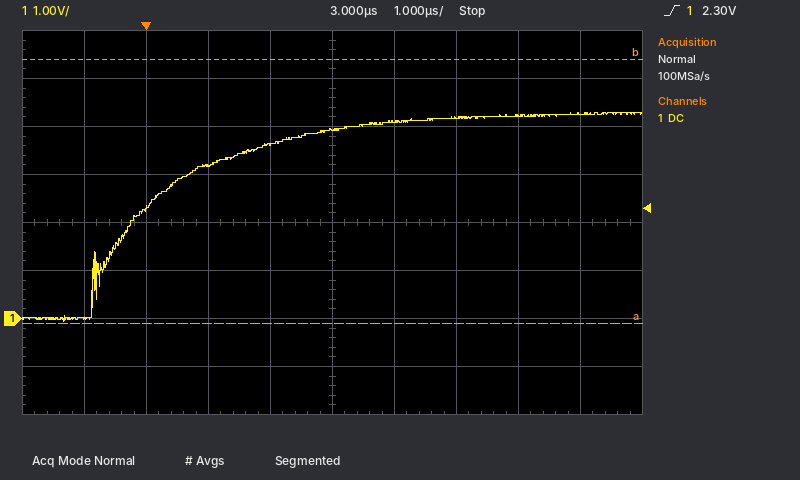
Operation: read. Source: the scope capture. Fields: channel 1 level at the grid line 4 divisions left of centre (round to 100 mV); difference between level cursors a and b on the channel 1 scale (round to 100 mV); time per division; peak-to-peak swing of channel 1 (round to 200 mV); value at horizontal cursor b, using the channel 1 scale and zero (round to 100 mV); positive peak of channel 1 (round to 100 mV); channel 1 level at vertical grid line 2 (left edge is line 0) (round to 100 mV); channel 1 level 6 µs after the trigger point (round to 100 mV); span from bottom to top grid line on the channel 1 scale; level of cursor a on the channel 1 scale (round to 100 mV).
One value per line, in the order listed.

0.0 V
5.5 V
1 µs
4.4 V
5.4 V
4.3 V
2.3 V
4.2 V
8 V
-100 mV
